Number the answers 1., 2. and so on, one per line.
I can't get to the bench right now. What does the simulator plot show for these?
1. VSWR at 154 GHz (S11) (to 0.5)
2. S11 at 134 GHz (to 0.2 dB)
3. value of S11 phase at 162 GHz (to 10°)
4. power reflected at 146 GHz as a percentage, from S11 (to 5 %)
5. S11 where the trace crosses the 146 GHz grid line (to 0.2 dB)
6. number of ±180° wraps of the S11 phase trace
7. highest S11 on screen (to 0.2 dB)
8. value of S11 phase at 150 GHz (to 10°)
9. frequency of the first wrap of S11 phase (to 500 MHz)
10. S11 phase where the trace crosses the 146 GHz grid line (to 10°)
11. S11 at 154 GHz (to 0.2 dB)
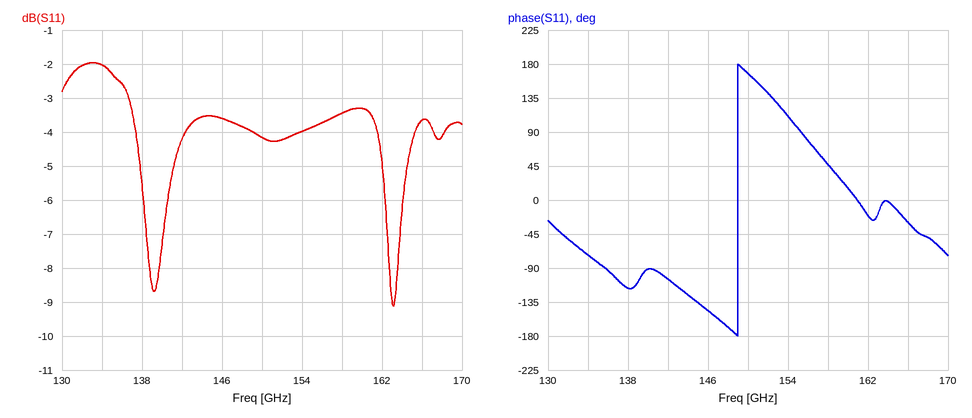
1. 4.5
2. -2.0 dB
3. -20°
4. 45 %
5. -3.6 dB
6. 1
7. -2.0 dB
8. 170°
9. 149.0 GHz
10. -150°
11. -4.0 dB
